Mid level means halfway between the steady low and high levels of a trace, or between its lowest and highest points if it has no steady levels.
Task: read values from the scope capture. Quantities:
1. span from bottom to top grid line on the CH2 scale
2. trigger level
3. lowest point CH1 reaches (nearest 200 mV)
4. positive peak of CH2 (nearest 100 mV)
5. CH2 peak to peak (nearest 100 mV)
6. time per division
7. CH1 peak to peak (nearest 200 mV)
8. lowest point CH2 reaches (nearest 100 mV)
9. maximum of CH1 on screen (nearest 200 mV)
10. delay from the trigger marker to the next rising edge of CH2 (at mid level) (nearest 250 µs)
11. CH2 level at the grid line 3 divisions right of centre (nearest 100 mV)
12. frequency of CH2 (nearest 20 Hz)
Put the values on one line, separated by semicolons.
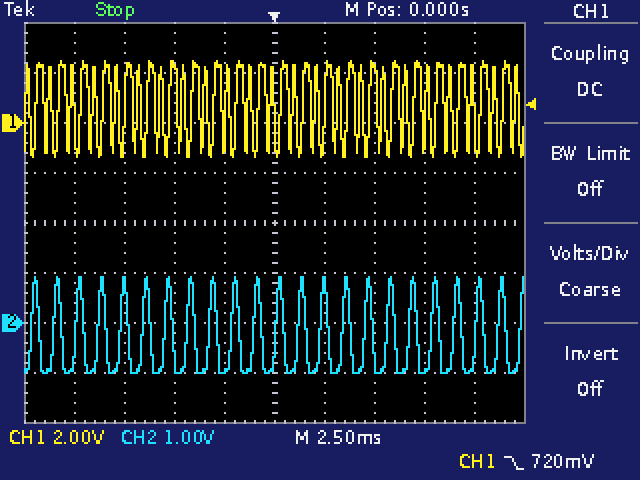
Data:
8 V; 720 mV; -1.4 V; 900 mV; 1.9 V; 2.5 ms; 3.8 V; -1.0 V; 2.4 V; 1.25 ms; -1.0 V; 900 Hz
